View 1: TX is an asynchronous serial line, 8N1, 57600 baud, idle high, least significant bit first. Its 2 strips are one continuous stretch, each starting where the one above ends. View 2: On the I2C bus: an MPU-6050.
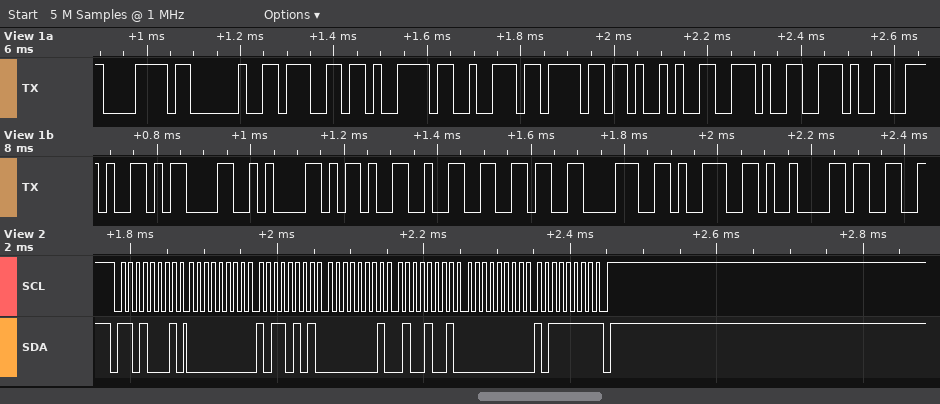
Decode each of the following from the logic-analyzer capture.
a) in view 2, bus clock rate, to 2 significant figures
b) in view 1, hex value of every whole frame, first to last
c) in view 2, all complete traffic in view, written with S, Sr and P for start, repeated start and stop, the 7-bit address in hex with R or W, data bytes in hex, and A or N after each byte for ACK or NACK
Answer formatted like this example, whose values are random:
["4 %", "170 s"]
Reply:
["100 kHz", "0x78 0x20 0x67 0x79 0x72 0x6F 0x29 0x2E 0x2E 0x2E 0x0D 0x0A 0x2D 0x32 0x36 0x38 0x39 0x09 0x33", "S 68R A 00 A B5 A 01 A 49 A 00 A BF N P"]
